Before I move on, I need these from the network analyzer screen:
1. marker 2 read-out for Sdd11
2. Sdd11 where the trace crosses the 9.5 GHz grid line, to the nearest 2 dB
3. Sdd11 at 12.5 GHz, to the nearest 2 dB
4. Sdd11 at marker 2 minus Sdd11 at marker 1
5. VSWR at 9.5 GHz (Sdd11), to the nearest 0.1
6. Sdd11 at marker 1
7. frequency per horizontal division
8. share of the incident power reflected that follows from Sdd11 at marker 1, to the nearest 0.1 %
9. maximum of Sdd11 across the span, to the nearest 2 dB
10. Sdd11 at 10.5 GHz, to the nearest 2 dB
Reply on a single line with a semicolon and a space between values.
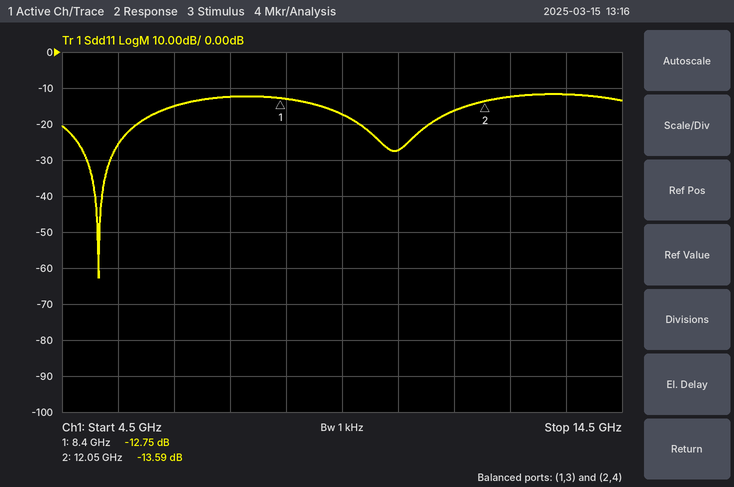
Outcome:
-13.59 dB; -18 dB; -12 dB; -0.84 dB; 1.3; -12.75 dB; 1 GHz; 5.3 %; -12 dB; -28 dB
